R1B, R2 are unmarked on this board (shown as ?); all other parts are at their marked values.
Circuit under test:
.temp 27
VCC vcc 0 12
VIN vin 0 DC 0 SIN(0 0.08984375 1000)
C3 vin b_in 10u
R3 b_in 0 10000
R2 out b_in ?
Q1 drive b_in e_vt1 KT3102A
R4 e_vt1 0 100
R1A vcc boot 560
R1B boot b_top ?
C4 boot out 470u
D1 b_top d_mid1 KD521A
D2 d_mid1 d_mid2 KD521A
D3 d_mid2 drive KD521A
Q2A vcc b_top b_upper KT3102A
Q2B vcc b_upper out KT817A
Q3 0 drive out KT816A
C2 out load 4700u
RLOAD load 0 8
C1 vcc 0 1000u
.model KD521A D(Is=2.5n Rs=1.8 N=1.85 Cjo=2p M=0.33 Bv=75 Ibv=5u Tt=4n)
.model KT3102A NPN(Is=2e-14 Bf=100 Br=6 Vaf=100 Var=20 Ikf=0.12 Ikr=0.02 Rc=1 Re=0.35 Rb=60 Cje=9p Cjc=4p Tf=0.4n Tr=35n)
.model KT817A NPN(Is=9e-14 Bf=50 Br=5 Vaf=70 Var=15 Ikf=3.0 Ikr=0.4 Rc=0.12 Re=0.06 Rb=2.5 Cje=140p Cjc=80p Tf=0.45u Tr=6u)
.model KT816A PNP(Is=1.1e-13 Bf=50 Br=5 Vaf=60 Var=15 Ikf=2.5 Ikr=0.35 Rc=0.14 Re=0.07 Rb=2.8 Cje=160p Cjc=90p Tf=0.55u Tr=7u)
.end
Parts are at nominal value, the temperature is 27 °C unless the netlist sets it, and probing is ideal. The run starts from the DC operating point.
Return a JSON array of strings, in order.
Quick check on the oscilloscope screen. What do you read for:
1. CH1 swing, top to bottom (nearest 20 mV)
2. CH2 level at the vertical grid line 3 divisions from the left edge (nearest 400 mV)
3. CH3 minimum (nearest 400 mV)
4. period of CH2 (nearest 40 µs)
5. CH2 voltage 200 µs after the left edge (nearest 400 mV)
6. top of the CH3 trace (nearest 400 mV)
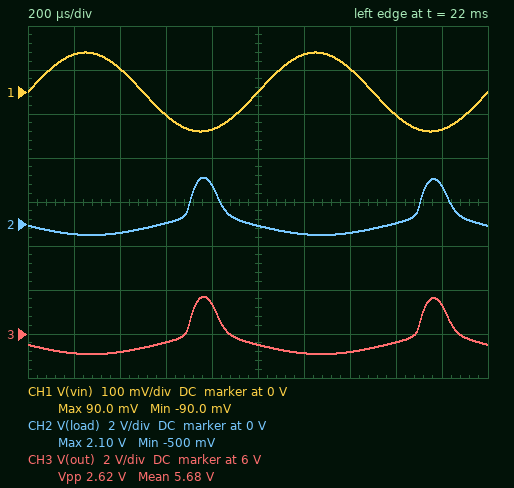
["180 mV", "0 V", "5.2 V", "1.00 ms", "-400 mV", "7.6 V"]
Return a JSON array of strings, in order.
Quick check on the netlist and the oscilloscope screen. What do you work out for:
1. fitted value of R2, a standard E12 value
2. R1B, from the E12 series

["39 kΩ", "2.2 kΩ"]
